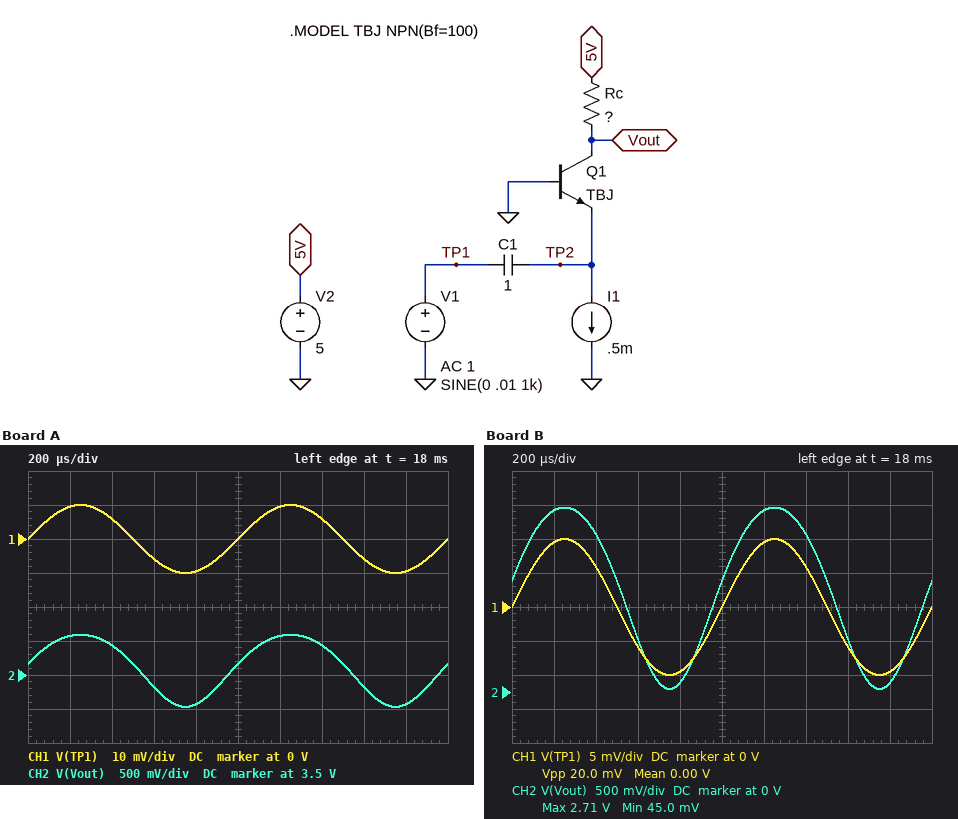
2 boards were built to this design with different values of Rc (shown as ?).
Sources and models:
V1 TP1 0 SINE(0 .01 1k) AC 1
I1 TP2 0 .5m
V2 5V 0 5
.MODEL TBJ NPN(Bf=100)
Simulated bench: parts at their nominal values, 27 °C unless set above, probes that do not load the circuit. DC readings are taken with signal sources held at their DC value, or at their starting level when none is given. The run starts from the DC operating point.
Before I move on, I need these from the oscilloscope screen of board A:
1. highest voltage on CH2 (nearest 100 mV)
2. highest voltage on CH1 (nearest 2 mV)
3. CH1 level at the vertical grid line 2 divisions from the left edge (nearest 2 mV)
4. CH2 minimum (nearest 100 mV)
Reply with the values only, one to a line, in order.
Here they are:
4.1 V
10 mV
6 mV
3.0 V
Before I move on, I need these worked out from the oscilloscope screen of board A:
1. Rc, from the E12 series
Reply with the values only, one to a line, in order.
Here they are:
2.7 kΩ
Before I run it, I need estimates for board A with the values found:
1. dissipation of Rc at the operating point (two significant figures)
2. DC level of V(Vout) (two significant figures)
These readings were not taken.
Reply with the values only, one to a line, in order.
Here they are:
660 µW
3.7 V
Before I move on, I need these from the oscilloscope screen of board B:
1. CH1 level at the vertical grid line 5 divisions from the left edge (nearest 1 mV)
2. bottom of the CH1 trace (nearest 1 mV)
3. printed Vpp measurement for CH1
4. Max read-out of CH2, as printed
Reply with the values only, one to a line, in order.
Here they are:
0 V
-10 mV
20.0 mV
2.71 V
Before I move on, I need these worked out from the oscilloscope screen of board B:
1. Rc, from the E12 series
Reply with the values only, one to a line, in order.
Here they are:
6.8 kΩ
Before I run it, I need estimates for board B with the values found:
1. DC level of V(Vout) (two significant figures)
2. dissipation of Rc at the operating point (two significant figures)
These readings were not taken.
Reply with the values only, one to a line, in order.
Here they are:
1.6 V
1.7 mW
